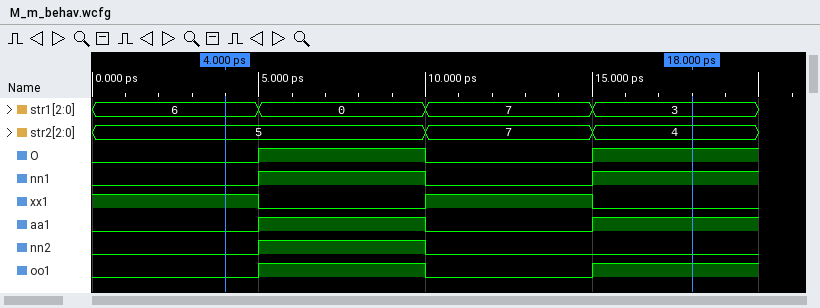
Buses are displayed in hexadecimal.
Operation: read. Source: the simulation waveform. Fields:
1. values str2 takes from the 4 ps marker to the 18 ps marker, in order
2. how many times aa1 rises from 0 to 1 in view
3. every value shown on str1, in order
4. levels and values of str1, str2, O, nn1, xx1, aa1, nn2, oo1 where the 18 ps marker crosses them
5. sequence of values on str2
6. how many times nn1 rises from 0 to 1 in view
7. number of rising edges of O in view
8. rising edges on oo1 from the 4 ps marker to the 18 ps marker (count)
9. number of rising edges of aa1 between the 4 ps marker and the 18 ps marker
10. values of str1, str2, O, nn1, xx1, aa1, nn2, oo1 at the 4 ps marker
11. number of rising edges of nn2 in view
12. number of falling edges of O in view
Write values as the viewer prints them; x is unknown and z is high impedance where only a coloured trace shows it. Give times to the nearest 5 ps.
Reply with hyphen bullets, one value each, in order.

- 5, 7, 4
- 2
- 6, 0, 7, 3
- str1=3, str2=4, O=1, nn1=1, xx1=0, aa1=1, nn2=0, oo1=1
- 5, 7, 4
- 2
- 2
- 2
- 2
- str1=6, str2=5, O=0, nn1=0, xx1=1, aa1=0, nn2=0, oo1=0
- 1
- 1
